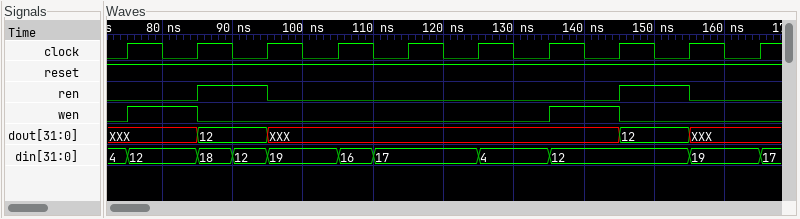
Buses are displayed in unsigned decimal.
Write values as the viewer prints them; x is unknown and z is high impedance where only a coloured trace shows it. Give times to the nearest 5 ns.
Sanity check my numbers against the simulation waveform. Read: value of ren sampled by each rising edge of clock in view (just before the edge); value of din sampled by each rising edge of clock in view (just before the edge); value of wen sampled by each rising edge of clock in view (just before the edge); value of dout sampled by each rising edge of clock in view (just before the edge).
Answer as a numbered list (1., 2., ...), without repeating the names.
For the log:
1. 0 0 1 0 0 0 0 0 1 0
2. 4, 12, 12, 19, 17, 17, 4, 12, 12, 19
3. 0 1 0 0 0 0 0 1 0 0
4. XXX, XXX, 12, XXX, XXX, XXX, XXX, XXX, 12, XXX
